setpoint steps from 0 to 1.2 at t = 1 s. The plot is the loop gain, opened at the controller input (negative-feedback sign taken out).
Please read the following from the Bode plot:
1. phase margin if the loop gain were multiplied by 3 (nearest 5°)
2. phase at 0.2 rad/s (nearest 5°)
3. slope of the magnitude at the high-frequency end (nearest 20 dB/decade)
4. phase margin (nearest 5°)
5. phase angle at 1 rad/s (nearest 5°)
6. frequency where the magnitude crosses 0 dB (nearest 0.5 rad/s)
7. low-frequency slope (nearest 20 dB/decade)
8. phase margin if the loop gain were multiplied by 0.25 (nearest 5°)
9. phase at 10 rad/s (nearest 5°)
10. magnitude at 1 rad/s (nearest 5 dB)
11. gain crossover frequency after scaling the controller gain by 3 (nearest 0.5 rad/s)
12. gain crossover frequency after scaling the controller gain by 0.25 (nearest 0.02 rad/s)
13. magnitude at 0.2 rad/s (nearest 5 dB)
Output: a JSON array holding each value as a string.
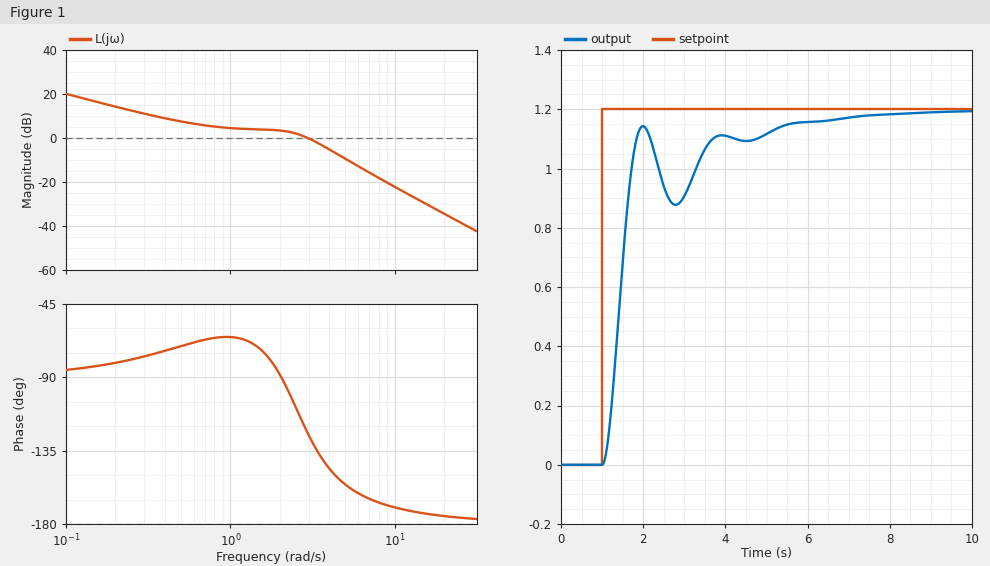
["25°", "-80°", "-40 dB/decade", "55°", "-65°", "3.0 rad/s", "-20 dB/decade", "100°", "-170°", "5 dB", "5.0 rad/s", "0.26 rad/s", "15 dB"]
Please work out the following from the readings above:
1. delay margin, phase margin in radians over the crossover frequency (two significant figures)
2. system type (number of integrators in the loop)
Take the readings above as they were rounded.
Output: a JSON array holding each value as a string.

["0.32 s", "1"]
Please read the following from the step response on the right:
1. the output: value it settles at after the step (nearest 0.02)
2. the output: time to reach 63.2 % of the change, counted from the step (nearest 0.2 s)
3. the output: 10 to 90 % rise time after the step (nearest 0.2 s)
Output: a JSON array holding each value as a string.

["1.20", "0.6 s", "0.6 s"]
